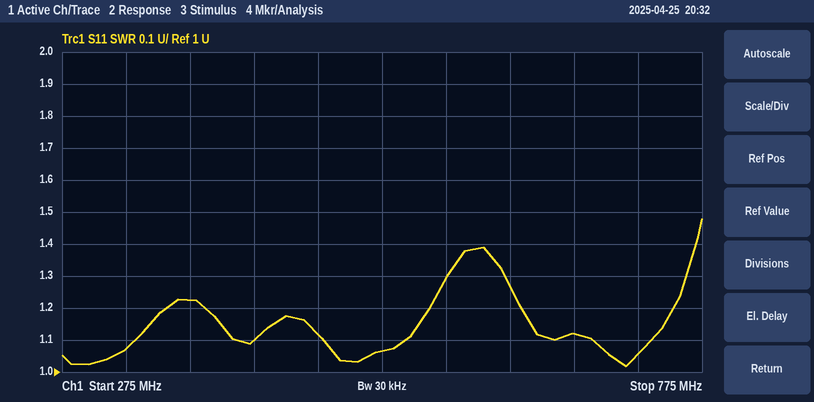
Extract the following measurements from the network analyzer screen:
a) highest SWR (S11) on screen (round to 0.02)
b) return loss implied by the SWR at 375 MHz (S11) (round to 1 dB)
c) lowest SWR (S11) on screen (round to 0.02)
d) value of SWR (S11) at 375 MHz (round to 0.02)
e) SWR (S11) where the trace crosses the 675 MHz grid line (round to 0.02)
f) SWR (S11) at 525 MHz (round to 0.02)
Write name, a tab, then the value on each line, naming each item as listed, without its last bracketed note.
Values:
highest SWR (S11) on screen	1.48
return loss implied by the SWR at 375 MHz (S11)	20 dB
lowest SWR (S11) on screen	1.02
value of SWR (S11) at 375 MHz	1.22
SWR (S11) where the trace crosses the 675 MHz grid line	1.12
SWR (S11) at 525 MHz	1.06
